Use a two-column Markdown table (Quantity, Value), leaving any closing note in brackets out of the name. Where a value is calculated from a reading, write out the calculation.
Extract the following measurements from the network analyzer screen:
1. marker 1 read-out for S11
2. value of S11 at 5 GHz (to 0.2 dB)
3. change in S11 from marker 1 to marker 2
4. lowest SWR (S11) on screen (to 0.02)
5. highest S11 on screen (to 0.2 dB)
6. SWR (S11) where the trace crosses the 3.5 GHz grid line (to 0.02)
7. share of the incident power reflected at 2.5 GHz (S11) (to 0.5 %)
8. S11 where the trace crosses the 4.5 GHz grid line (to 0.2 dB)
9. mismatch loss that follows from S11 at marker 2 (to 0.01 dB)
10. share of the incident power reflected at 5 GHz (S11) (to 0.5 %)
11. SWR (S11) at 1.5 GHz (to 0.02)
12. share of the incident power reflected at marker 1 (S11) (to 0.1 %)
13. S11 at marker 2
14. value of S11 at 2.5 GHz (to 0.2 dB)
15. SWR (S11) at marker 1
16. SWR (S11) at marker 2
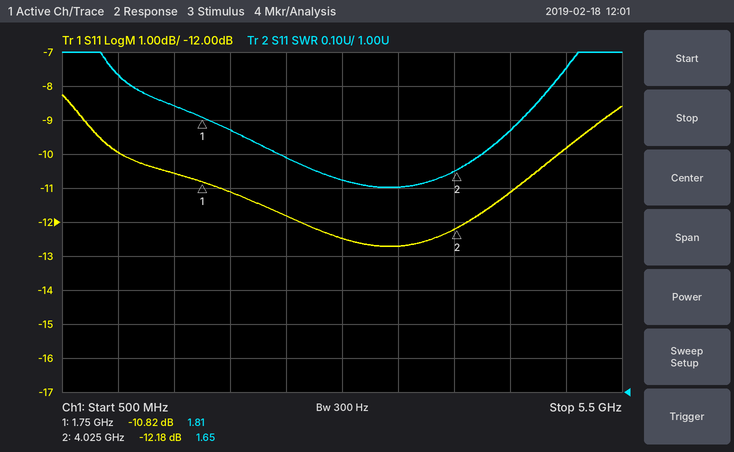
| Quantity | Value |
|---|---|
| marker 1 read-out for S11 | -10.82 dB |
| value of S11 at 5 GHz | -9.8 dB |
| change in S11 from marker 1 to marker 2 | -12.18 − (-10.82) = -1.36 dB |
| lowest SWR (S11) on screen | 1.60 |
| highest S11 on screen | -8.2 dB |
| SWR (S11) where the trace crosses the 3.5 GHz grid line | 1.60 |
| share of the incident power reflected at 2.5 GHz (S11) | 10^(-11.8/10) ≈ 6.61 %, so 6.5 % to the nearest 0.5 % |
| S11 where the trace crosses the 4.5 GHz grid line | -11.2 dB |
| mismatch loss that follows from S11 at marker 2 | −10 log10(1 − 10^(-12.18/10)) ≈ 0.27 dB |
| share of the incident power reflected at 5 GHz (S11) | 10^(-9.8/10) ≈ 10.5 % |
| SWR (S11) at 1.5 GHz | 1.84 |
| share of the incident power reflected at marker 1 (S11) | 10^(-10.82/10) ≈ 8.3 % |
| S11 at marker 2 | -12.18 dB |
| value of S11 at 2.5 GHz | -11.8 dB |
| SWR (S11) at marker 1 | 1.81 |
| SWR (S11) at marker 2 | 1.65 |
